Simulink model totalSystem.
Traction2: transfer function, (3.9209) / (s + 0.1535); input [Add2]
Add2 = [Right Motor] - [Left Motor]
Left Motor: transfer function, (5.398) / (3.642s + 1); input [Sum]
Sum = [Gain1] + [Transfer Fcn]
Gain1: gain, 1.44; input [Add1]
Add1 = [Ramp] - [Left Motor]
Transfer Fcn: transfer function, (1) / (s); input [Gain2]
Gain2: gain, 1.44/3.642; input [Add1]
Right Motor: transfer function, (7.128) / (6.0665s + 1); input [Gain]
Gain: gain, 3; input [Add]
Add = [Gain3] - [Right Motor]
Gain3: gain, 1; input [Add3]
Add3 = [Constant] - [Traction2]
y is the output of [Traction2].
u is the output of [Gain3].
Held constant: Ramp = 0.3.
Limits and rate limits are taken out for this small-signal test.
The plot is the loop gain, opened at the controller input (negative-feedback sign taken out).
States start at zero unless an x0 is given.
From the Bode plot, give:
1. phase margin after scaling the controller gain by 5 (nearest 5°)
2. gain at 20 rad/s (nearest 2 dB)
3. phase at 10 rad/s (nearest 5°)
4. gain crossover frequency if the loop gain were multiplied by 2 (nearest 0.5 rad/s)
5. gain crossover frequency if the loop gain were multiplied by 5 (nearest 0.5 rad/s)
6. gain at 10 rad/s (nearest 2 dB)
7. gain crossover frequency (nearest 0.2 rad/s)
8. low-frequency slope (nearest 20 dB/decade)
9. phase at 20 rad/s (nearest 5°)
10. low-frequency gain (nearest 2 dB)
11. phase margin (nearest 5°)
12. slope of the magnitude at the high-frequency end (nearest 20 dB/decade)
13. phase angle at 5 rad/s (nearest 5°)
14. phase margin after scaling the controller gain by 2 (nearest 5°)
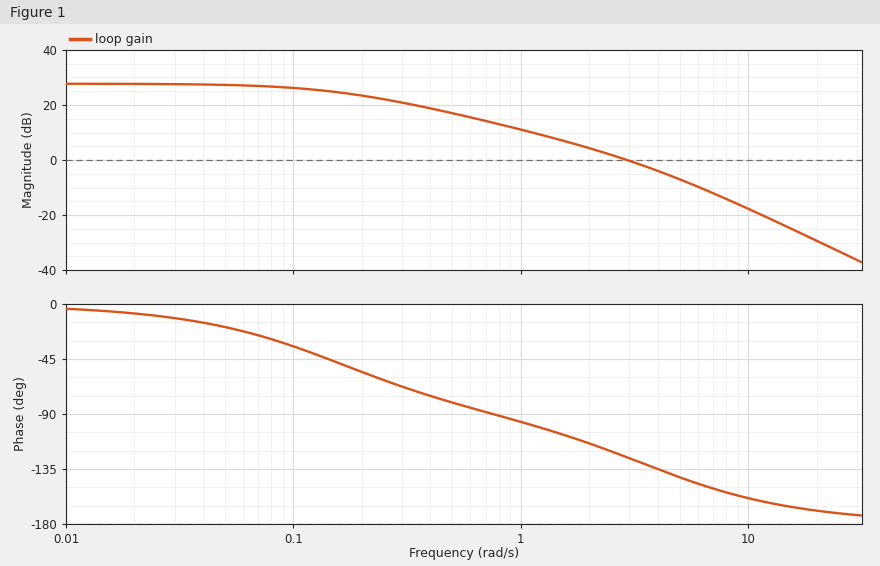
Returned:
25°
-30 dB
-160°
4.5 rad/s
8.0 rad/s
-18 dB
3.0 rad/s
0 dB/decade
-170°
28 dB
55°
-40 dB/decade
-140°
40°
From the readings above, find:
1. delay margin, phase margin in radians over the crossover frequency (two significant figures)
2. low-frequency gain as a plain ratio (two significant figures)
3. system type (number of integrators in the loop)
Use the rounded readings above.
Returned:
0.32 s
25
0
